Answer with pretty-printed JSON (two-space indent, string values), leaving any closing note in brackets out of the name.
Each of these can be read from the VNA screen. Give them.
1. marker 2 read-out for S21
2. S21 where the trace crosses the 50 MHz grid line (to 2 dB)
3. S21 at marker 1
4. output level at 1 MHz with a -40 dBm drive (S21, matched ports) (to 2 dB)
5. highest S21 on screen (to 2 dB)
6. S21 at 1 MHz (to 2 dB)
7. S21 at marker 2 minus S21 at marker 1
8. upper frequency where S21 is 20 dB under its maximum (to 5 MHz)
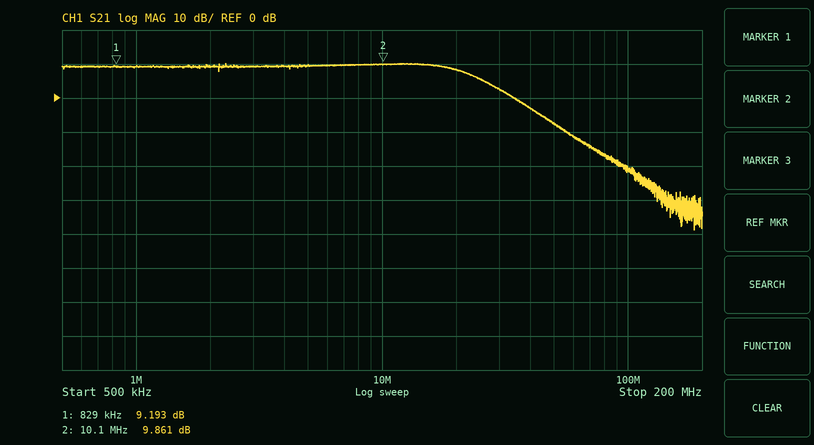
{
  "marker 2 read-out for S21": "9.861 dB",
  "S21 where the trace crosses the 50 MHz grid line": "-8 dB",
  "S21 at marker 1": "9.193 dB",
  "output level at 1 MHz with a -40 dBm drive (S21, matched ports)": "-30 dBm",
  "highest S21 on screen": "10 dB",
  "S21 at 1 MHz": "10 dB",
  "S21 at marker 2 minus S21 at marker 1": "0.668 dB",
  "upper frequency where S21 is 20 dB under its maximum": "55 MHz"
}
